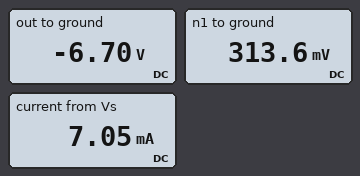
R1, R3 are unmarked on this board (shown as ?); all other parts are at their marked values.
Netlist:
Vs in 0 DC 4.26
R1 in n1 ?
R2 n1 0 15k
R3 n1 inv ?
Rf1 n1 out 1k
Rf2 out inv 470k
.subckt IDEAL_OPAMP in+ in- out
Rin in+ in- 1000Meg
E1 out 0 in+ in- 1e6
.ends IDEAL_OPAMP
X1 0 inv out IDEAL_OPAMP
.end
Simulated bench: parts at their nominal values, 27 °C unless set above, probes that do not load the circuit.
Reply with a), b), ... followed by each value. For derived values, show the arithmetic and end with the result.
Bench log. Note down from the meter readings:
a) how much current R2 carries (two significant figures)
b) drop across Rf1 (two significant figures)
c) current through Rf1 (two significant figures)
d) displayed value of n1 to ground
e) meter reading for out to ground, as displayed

a) (313.6 mV) / 15 kΩ = 21 µA
b) 313.6 mV - (-6.7 V) = 7.0 V
c) (313.6 mV - (-6.7 V)) / 1 kΩ = 7.0 mA
d) 313.6 mV
e) -6.70 V
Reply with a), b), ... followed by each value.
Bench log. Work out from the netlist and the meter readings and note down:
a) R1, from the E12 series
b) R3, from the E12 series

a) 560 Ω
b) 22 kΩ
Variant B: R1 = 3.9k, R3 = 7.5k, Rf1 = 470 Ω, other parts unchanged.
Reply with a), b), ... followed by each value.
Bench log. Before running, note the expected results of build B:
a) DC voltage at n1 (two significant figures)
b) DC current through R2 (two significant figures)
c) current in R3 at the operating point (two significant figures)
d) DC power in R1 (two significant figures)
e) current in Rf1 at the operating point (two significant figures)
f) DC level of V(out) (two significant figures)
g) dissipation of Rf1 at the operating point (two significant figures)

a) 8.0 mV
b) 540 nA
c) 1.1 µA
d) 4.6 mW
e) 1.1 mA
f) -500 mV
g) 560 µW
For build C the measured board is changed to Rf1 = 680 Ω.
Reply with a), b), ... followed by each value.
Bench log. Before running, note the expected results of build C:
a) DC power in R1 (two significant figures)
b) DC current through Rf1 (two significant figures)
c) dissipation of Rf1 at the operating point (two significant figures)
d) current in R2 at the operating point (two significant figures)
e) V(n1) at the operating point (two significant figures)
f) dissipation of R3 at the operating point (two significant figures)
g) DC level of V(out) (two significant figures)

a) 29 mW
b) 7.2 mA
c) 35 mW
d) 15 µA
e) 220 mV
f) 2.2 µW
g) -4.7 V
